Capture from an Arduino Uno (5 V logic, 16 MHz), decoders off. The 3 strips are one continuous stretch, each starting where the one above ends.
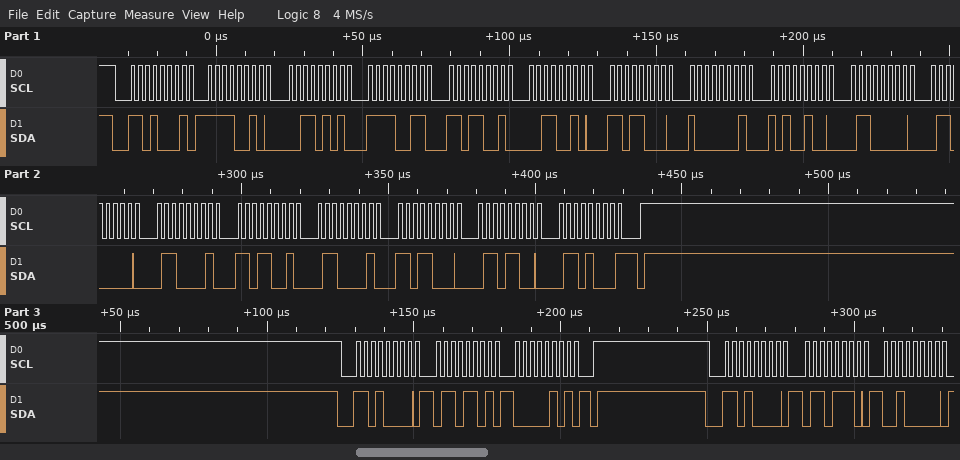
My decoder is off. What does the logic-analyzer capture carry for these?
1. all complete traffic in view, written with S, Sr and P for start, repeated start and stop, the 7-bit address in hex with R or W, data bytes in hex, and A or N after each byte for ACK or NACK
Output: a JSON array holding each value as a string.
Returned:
["S 68R A F2 A 35 A F3 A D9 A 32 A D8 A 81 A A4 A 60 A 60 A 61 A D9 A 61 A D8 A 6C A 68 N P S 68W A 6D A 05 A P S 68W A 6E A 20 A"]
